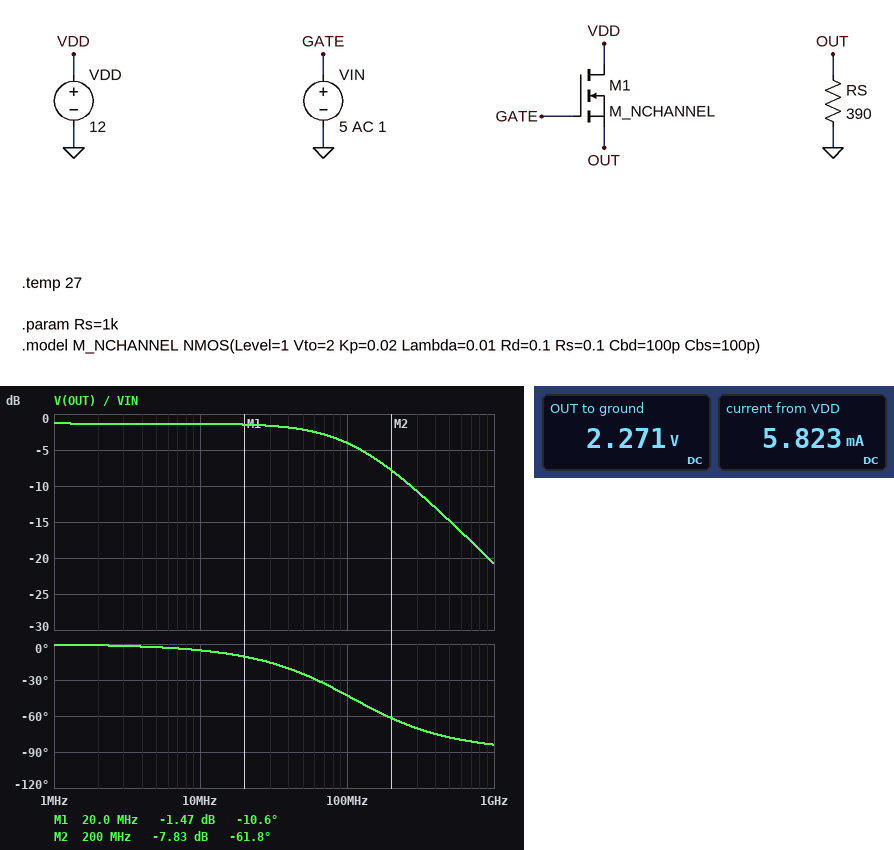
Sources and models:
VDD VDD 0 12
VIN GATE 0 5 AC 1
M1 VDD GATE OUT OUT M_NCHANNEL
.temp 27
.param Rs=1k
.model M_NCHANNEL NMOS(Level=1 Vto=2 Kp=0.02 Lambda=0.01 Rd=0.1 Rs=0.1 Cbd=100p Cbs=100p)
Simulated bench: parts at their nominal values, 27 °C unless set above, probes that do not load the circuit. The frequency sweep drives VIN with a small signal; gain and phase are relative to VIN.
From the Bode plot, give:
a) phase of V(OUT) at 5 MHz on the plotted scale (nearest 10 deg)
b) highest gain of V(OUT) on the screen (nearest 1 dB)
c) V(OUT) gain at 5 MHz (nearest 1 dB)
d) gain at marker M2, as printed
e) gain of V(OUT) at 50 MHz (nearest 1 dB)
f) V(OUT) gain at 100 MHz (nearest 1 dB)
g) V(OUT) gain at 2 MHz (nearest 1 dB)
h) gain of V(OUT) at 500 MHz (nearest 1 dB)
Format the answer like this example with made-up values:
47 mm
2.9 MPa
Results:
0 deg
-1 dB
-1 dB
-7.83 dB
-2 dB
-4 dB
-1 dB
-15 dB
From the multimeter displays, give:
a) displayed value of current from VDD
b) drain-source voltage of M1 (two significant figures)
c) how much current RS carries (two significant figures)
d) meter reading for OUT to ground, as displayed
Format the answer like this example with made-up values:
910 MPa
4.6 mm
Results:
5.823 mA
9.7 V
5.8 mA
2.271 V
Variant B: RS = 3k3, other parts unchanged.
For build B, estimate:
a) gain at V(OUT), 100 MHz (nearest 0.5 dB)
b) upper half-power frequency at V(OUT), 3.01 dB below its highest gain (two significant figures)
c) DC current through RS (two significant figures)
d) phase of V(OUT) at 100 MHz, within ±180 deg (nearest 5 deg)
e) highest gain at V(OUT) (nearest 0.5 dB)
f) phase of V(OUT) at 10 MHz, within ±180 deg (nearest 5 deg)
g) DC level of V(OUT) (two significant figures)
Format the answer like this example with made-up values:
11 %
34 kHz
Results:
-10.0 dB
36 MHz
830 µA
-70 deg
-0.5 dB
-15 deg
2.7 V
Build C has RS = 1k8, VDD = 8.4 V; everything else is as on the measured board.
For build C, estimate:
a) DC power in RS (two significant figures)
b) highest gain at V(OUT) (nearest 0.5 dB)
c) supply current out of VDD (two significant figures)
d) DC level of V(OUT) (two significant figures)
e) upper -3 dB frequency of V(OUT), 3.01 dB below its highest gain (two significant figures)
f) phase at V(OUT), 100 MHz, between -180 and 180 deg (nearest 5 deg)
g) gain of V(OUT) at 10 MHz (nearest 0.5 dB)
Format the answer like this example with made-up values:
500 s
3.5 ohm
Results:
3.8 mW
-0.5 dB
1.5 mA
2.6 V
38 MHz
-70 deg
-1.0 dB
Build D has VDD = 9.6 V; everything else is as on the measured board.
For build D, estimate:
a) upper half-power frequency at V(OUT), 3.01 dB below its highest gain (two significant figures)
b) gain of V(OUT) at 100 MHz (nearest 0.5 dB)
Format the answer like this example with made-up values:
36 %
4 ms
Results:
93 MHz
-4.5 dB
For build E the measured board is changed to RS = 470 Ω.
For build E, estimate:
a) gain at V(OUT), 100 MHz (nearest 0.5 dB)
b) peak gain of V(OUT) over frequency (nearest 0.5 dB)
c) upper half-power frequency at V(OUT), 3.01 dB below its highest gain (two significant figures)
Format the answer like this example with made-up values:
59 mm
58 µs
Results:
-4.5 dB
-1.0 dB
97 MHz
